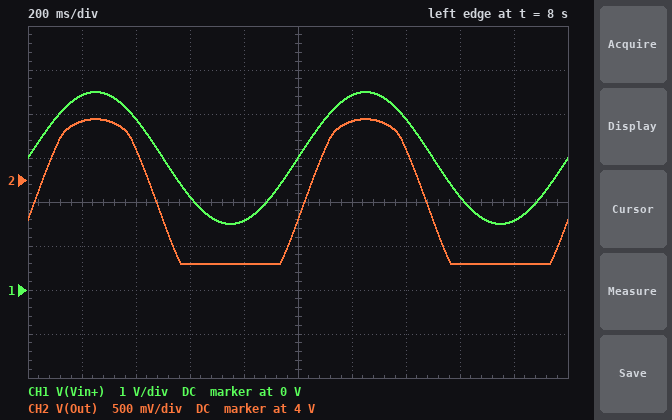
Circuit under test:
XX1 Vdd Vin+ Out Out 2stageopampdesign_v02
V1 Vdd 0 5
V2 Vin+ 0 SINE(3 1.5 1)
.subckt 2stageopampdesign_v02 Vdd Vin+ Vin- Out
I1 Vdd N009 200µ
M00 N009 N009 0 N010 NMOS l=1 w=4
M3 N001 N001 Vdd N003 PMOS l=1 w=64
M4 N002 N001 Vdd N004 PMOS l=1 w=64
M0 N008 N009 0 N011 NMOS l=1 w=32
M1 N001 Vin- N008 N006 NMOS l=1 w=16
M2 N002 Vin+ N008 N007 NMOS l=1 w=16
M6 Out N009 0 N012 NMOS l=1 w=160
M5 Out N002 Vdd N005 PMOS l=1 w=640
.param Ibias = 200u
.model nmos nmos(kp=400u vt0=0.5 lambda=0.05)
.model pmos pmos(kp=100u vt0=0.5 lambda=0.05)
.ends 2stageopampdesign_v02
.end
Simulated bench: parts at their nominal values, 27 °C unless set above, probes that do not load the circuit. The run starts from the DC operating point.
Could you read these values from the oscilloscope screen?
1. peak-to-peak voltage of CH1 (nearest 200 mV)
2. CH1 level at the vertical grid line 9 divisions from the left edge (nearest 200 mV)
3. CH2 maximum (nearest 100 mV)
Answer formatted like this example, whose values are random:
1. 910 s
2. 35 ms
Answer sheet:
1. 3.0 V
2. 1.6 V
3. 4.7 V
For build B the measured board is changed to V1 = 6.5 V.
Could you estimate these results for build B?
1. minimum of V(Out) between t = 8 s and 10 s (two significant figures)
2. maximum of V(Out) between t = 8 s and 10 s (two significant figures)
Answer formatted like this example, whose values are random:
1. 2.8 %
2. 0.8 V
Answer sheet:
1. 3.8 V
2. 5.0 V
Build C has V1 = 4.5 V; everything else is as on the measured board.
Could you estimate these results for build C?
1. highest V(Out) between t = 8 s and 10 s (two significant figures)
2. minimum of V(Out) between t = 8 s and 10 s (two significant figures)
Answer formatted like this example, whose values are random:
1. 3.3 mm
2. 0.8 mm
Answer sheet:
1. 4.3 V
2. 2.8 V
